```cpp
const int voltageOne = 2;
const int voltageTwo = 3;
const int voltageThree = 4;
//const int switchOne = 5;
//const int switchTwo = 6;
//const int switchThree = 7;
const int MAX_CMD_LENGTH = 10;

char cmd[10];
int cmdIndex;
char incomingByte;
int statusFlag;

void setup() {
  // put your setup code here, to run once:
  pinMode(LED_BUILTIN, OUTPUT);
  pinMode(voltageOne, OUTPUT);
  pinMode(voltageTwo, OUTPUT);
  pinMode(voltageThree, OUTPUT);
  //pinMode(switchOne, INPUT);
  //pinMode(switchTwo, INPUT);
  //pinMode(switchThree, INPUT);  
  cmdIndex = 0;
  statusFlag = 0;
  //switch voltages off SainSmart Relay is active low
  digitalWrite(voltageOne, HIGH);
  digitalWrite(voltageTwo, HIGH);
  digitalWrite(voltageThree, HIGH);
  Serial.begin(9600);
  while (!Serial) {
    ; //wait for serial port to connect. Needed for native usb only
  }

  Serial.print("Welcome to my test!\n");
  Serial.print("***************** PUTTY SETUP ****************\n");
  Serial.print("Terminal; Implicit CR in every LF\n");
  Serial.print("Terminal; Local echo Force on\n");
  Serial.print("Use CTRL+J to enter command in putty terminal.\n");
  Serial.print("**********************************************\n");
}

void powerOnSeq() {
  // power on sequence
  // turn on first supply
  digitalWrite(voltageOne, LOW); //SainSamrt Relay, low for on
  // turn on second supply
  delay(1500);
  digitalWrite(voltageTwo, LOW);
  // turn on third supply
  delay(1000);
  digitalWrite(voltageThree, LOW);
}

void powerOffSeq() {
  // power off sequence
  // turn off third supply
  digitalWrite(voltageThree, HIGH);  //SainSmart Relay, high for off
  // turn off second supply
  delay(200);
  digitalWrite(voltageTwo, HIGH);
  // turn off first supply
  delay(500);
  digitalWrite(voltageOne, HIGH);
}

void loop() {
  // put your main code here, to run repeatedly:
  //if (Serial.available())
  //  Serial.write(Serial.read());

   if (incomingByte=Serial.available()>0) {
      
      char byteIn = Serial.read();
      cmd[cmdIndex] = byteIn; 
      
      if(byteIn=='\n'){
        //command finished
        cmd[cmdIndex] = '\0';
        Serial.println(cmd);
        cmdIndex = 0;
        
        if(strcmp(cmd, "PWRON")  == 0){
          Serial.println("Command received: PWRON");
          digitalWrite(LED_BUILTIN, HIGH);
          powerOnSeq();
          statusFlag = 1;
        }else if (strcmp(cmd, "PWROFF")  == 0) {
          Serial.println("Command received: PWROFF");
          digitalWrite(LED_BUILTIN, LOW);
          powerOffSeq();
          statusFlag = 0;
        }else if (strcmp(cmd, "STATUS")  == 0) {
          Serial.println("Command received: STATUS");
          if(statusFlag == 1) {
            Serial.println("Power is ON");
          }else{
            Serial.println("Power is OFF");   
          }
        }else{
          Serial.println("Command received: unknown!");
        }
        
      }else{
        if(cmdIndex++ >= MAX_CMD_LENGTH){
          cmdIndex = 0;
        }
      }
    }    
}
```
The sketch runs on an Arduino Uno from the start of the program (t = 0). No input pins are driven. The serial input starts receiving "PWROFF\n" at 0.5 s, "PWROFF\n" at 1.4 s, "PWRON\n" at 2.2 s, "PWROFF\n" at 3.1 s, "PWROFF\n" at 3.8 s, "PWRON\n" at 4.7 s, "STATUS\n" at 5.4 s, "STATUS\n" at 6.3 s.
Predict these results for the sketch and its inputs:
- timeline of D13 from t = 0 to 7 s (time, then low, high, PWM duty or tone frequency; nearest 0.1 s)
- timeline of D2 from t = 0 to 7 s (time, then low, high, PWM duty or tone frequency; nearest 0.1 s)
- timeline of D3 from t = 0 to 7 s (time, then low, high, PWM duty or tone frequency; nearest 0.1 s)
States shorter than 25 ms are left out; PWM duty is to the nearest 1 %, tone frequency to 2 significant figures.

0 s low; 2.2 s high; 4.7 s low; 6.1 s high
0 s high; 2.2 s low; 5.4 s high; 6.1 s low
0 s high; 3.7 s low; 4.9 s high
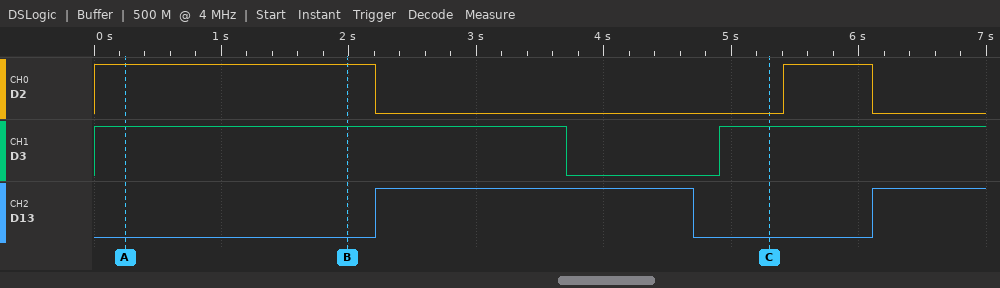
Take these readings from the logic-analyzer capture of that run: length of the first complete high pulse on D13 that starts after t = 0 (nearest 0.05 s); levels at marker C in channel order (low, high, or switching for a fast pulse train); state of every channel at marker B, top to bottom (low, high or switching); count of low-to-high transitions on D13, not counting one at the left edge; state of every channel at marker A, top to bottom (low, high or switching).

2.50 s
D2 low, D3 high, D13 low
D2 high, D3 high, D13 low
2
D2 high, D3 high, D13 low
